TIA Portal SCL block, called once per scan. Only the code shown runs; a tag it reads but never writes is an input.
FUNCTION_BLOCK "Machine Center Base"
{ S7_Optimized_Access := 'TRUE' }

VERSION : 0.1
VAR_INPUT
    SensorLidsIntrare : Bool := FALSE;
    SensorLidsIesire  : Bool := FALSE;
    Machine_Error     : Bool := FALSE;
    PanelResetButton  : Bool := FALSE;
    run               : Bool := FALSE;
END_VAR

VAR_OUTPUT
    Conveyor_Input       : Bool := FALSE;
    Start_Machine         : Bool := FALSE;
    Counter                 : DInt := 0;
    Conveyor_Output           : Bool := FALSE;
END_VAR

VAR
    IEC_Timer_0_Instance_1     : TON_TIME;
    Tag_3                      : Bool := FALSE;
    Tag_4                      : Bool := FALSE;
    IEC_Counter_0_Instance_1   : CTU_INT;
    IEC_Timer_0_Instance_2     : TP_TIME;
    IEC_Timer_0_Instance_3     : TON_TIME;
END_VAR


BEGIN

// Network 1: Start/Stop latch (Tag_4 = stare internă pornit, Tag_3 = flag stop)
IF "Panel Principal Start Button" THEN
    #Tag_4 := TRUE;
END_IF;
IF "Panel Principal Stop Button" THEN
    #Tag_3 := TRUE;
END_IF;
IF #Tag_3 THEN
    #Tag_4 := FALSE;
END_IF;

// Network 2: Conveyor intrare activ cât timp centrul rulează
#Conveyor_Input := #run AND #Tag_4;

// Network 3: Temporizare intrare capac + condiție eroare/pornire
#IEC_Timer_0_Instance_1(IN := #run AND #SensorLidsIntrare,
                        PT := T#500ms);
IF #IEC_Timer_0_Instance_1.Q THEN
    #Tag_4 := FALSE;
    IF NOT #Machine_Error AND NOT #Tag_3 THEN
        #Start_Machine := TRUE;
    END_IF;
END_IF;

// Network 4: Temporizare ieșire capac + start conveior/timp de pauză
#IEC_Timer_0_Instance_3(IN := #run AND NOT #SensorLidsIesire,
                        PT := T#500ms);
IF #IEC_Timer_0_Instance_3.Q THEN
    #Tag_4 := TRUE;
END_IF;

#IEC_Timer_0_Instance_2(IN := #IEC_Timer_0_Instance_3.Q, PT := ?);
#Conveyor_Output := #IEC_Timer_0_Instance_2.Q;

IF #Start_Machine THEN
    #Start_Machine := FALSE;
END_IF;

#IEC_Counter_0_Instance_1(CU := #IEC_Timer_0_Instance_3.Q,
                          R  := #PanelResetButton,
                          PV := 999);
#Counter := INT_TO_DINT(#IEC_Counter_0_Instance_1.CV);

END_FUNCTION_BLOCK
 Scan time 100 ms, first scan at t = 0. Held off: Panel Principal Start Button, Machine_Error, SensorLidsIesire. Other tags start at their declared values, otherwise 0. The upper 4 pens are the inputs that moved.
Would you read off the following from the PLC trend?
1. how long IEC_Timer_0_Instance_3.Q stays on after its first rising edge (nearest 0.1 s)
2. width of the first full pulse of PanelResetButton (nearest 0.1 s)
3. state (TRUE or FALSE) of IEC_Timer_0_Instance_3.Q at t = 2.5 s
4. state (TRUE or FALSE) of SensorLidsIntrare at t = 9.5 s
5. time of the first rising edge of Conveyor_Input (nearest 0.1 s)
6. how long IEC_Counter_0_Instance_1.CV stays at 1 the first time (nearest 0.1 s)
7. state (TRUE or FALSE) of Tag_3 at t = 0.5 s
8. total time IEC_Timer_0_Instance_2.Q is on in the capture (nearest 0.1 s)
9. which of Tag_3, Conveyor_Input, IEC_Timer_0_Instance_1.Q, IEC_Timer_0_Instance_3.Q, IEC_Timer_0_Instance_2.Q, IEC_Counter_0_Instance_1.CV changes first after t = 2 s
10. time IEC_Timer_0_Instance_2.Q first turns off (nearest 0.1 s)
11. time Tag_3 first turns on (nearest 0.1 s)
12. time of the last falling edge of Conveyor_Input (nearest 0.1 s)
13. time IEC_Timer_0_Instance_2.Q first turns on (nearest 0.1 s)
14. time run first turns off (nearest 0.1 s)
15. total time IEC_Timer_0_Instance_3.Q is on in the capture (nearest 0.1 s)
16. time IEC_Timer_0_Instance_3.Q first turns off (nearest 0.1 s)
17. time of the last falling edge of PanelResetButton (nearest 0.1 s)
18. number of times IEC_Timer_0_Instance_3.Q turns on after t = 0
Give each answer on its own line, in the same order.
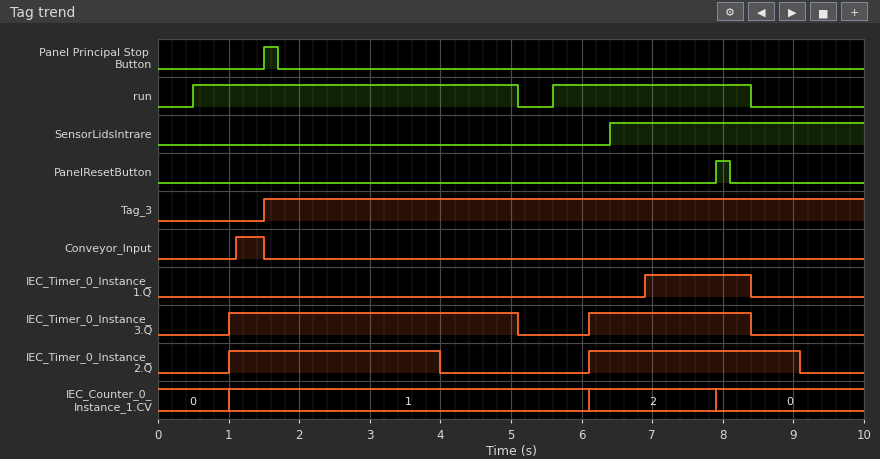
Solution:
4.1 s
0.2 s
TRUE
TRUE
1.1 s
5.1 s
FALSE
6.0 s
IEC_Timer_0_Instance_2.Q
4.0 s
1.5 s
1.5 s
1.0 s
5.1 s
6.4 s
5.1 s
8.1 s
2
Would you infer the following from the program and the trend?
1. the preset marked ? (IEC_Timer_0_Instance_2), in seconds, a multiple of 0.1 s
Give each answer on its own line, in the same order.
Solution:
3.0 s
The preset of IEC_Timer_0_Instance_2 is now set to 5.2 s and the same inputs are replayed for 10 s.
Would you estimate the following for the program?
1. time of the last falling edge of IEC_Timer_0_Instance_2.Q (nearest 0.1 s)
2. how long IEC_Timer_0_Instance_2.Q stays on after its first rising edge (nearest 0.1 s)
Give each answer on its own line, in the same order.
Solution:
6.2 s
5.2 s
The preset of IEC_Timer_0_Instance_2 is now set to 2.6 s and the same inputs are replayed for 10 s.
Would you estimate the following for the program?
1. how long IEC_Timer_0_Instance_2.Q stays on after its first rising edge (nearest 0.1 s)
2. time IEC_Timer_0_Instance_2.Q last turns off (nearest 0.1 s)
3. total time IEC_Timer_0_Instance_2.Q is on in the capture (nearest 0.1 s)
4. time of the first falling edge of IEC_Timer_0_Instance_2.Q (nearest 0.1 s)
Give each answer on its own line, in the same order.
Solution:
2.6 s
8.7 s
5.2 s
3.6 s
